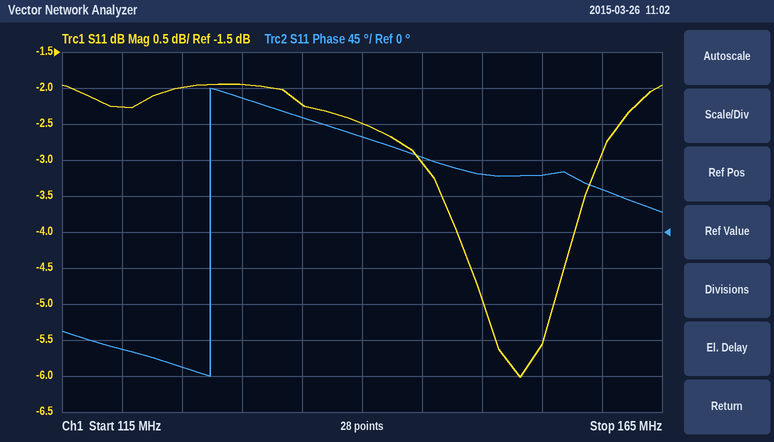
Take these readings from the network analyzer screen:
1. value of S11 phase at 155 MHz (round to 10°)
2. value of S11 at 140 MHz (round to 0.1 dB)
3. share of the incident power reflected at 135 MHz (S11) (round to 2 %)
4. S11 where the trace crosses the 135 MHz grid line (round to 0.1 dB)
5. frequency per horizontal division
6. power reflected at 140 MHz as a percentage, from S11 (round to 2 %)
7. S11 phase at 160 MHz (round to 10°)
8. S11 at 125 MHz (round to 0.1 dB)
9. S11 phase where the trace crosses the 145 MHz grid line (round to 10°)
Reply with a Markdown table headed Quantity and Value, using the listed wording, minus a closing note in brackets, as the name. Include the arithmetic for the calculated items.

| Quantity | Value |
|---|---|
| value of S11 phase at 155 MHz | 70° |
| value of S11 at 140 MHz | -2.5 dB |
| share of the incident power reflected at 135 MHz (S11) | 10^(-2.2/10) ≈ 60 % |
| S11 where the trace crosses the 135 MHz grid line | -2.2 dB |
| frequency per horizontal division | 5 MHz |
| power reflected at 140 MHz as a percentage, from S11 | 10^(-2.5/10) ≈ 56 % |
| S11 phase at 160 MHz | 50° |
| S11 at 125 MHz | -2.0 dB |
| S11 phase where the trace crosses the 145 MHz grid line | 90° |
